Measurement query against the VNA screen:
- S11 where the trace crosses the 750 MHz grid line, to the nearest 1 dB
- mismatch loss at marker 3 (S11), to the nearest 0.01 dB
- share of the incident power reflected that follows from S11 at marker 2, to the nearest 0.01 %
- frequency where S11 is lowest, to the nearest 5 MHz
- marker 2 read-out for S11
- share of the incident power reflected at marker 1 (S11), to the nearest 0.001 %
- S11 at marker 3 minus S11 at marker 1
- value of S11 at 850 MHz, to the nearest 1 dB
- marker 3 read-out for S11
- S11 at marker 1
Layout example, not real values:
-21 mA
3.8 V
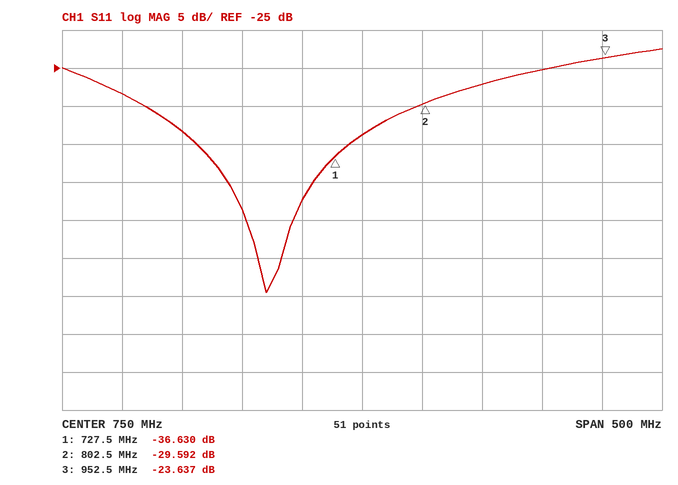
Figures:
-34 dB
0.02 dB
0.11 %
670 MHz
-29.592 dB
0.022 %
12.993 dB
-27 dB
-23.637 dB
-36.630 dB
